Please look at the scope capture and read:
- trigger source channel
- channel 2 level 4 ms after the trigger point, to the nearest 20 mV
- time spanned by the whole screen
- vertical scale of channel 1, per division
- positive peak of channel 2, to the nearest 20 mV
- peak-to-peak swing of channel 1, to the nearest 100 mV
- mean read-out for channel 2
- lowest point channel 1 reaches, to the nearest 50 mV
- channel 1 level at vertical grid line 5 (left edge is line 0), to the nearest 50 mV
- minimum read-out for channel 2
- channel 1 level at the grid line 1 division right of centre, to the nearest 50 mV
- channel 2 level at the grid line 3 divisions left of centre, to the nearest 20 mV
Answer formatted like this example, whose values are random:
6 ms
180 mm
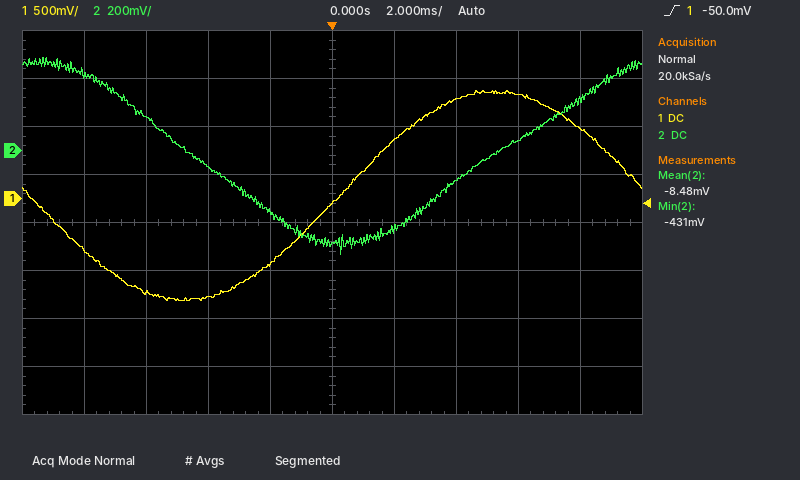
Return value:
channel 1
-120 mV
20 ms
500 mV
380 mV
2.20 V
-8.48 mV
-1.05 V
-50 mV
-431 mV
600 mV
140 mV
